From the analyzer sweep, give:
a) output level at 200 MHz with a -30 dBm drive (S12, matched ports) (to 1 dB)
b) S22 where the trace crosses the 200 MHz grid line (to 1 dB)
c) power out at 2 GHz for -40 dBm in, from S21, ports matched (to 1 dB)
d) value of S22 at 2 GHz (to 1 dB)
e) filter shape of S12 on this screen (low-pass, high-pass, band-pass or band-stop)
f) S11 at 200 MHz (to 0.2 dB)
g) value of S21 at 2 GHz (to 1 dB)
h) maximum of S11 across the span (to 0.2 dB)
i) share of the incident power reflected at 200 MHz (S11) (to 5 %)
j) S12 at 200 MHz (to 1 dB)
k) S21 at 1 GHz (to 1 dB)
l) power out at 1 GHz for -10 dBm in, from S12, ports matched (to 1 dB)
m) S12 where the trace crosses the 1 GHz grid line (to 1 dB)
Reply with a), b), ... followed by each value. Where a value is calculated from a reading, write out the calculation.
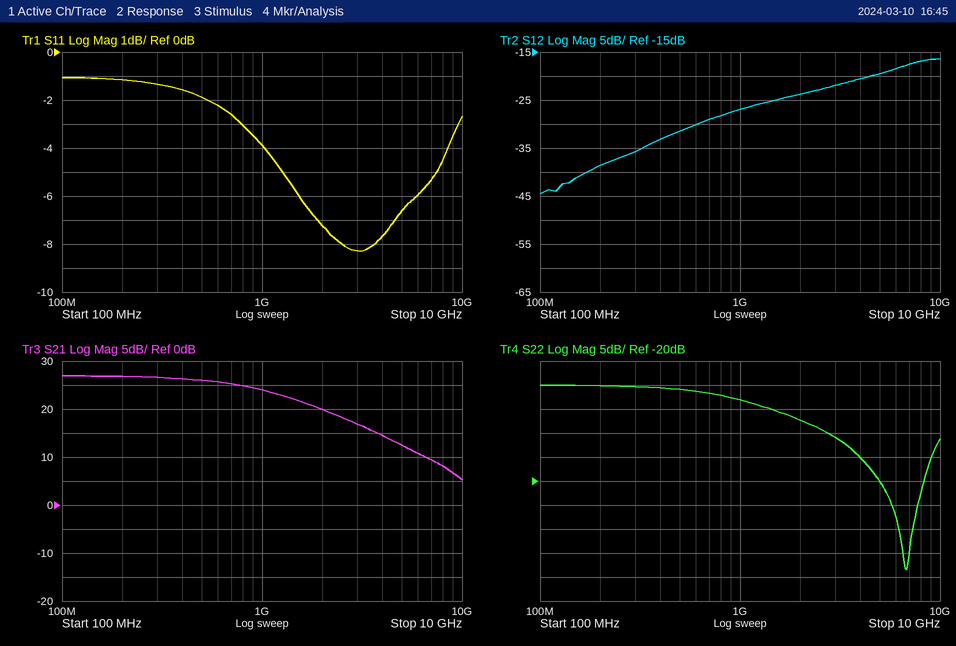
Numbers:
a) -30 dBm + (-39 dB) = -69 dBm
b) 0 dB
c) -40 dBm + (20 dB) = -20 dBm
d) -7 dB
e) high-pass
f) -1.2 dB
g) 20 dB
h) -1.0 dB
i) 10^(-1.2/10) ≈ 75.9 %, so 75 % to the nearest 5 %
j) -39 dB
k) 24 dB
l) -10 dBm + (-27 dB) = -37 dBm
m) -27 dB
